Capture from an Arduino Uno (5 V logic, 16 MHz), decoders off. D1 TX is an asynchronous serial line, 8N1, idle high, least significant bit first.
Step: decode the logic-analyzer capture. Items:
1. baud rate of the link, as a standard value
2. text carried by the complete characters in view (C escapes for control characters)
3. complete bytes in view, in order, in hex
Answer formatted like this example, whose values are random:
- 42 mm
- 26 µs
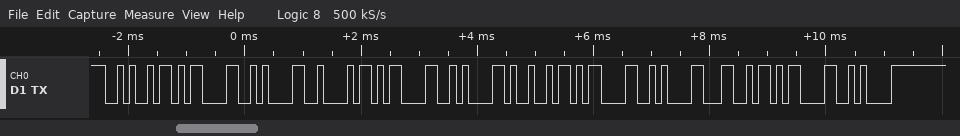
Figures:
- 9600 baud
- "J\r\nB\r\nI\r\nL\r\n"
- 0x4A 0x0D 0x0A 0x42 0x0D 0x0A 0x49 0x0D 0x0A 0x4C 0x0D 0x0A
